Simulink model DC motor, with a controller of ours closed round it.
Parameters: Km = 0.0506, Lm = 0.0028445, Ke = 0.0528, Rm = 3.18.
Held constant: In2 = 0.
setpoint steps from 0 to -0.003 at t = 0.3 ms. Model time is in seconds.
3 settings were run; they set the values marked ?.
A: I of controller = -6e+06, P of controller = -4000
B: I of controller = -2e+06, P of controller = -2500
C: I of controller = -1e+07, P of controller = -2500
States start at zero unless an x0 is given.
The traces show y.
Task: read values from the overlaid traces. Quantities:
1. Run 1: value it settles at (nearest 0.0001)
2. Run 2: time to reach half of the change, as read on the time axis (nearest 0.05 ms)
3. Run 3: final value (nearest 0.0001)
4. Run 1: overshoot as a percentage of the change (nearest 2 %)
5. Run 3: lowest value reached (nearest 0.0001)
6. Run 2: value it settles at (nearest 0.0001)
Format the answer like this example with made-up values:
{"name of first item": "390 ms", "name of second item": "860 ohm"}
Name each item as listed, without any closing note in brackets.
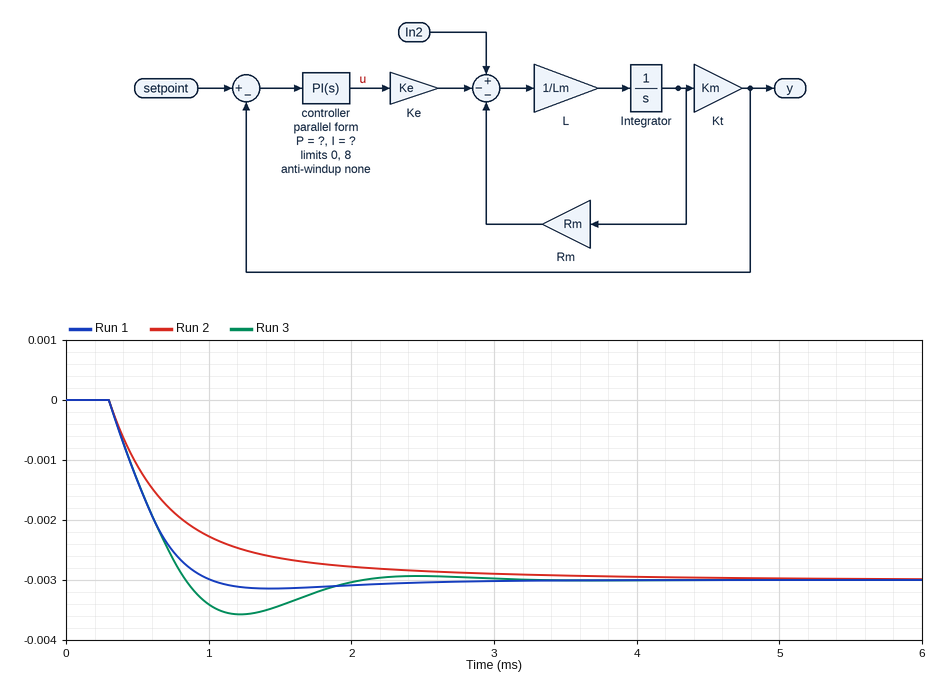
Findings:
{"Run 1: value it settles at": "-0.0030", "Run 2: time to reach half of the change, as read on the time axis": "0.60 ms", "Run 3: final value": "-0.0030", "Run 1: overshoot as a percentage of the change": "4 %", "Run 3: lowest value reached": "-0.0036", "Run 2: value it settles at": "-0.0030"}
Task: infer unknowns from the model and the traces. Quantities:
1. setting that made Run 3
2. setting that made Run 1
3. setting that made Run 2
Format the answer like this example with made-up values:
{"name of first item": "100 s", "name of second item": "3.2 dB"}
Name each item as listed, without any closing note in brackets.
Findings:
{"setting that made Run 3": "C", "setting that made Run 1": "A", "setting that made Run 2": "B"}
